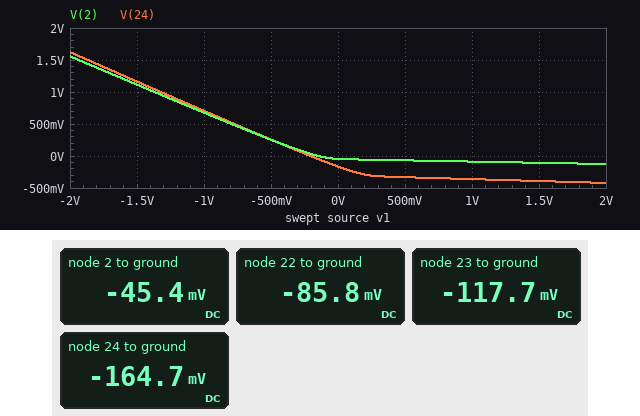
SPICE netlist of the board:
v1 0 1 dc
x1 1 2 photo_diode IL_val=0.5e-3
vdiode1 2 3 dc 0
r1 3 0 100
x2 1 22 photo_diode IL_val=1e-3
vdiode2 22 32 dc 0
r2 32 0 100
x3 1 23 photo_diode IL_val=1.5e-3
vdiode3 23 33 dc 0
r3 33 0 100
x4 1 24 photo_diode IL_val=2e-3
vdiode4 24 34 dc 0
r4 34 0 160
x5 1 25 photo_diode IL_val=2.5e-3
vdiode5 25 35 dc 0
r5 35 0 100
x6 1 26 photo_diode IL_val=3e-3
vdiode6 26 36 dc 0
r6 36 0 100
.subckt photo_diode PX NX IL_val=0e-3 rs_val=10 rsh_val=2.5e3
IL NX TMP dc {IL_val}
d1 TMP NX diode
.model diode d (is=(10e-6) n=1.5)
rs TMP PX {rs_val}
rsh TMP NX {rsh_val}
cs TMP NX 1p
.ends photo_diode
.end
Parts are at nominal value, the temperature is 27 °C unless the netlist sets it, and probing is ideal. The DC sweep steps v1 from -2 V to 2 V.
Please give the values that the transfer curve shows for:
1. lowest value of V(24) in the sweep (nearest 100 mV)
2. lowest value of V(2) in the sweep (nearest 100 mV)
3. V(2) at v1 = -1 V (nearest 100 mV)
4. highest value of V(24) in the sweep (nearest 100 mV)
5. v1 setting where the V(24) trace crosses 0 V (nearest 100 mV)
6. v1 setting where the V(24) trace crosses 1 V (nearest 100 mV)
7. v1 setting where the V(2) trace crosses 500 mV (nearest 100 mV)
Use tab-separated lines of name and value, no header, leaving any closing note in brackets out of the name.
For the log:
lowest value of V(24) in the sweep	-400 mV
lowest value of V(2) in the sweep	-100 mV
V(2) at v1 = -1 V	700 mV
highest value of V(24) in the sweep	1.6 V
v1 setting where the V(24) trace crosses 0 V	-200 mV
v1 setting where the V(24) trace crosses 1 V	-1.3 V
v1 setting where the V(2) trace crosses 500 mV	-800 mV
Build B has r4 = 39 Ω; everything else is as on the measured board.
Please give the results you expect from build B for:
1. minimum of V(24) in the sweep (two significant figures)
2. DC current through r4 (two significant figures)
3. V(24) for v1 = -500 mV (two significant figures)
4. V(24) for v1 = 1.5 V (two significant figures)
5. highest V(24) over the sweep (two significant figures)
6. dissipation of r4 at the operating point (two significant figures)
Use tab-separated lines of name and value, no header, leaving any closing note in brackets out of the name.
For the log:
minimum of V(24) in the sweep	-110 mV
DC current through r4	1.9 mA
V(24) for v1 = -500 mV	200 mV
V(24) for v1 = 1.5 V	-100 mV
highest V(24) over the sweep	1.3 V
dissipation of r4 at the operating point	140 µW
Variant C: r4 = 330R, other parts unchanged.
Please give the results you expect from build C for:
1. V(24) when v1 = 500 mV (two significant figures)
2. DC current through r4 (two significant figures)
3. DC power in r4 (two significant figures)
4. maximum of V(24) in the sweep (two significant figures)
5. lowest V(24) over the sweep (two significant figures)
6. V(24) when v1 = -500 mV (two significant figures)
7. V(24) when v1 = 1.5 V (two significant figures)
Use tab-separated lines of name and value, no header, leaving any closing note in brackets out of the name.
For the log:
V(24) when v1 = 500 mV	-590 mV
DC current through r4	560 µA
DC power in r4	100 µW
maximum of V(24) in the sweep	1.7 V
lowest V(24) over the sweep	-820 mV
V(24) when v1 = -500 mV	270 mV
V(24) when v1 = 1.5 V	-760 mV
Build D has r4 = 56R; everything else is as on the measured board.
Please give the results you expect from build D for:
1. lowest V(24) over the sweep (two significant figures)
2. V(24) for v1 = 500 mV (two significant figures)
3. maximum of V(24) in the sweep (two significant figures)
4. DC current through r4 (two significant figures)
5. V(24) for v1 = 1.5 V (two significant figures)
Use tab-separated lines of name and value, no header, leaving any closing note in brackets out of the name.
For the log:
lowest V(24) over the sweep	-150 mV
V(24) for v1 = 500 mV	-120 mV
maximum of V(24) in the sweep	1.4 V
DC current through r4	1.8 mA
V(24) for v1 = 1.5 V	-140 mV
